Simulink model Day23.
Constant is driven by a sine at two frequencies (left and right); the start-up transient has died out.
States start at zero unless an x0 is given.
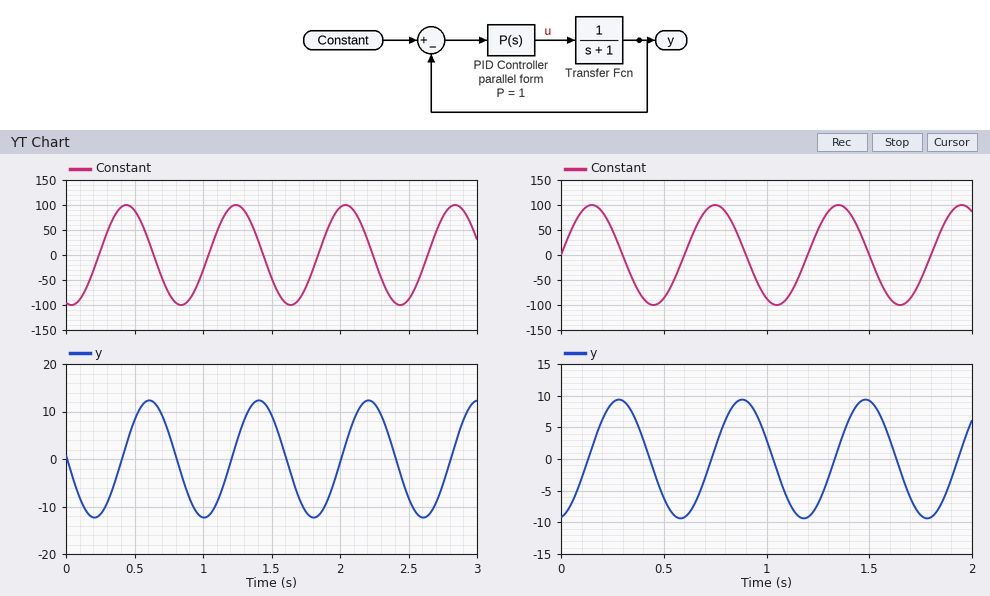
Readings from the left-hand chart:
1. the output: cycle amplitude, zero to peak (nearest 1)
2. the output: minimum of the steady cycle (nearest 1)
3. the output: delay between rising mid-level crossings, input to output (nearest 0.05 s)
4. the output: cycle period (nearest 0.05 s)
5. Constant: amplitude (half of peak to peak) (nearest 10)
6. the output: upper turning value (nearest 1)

12
-12
0.15 s
0.80 s
100
12
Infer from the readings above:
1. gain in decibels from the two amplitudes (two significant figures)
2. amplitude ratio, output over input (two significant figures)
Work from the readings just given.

-18 dB
0.12
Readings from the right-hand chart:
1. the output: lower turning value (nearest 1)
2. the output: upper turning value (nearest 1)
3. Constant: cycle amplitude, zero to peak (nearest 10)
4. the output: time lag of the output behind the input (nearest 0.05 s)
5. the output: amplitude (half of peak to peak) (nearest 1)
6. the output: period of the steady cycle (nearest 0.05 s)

-9
9
100
0.15 s
9
0.60 s
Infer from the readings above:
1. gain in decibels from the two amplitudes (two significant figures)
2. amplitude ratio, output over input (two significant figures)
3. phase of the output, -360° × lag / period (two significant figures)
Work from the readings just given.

-21 dB
0.090
-90°
